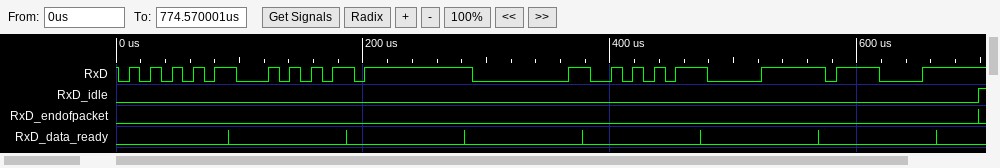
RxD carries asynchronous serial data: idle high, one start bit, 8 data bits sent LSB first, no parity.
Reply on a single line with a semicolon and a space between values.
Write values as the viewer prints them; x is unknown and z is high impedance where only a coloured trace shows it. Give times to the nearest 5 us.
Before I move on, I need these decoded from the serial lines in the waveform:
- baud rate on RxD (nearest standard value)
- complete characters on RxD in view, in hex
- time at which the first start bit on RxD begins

115200 baud; 55, 54, FF, 00, AA, F0, 0F; 0 us
